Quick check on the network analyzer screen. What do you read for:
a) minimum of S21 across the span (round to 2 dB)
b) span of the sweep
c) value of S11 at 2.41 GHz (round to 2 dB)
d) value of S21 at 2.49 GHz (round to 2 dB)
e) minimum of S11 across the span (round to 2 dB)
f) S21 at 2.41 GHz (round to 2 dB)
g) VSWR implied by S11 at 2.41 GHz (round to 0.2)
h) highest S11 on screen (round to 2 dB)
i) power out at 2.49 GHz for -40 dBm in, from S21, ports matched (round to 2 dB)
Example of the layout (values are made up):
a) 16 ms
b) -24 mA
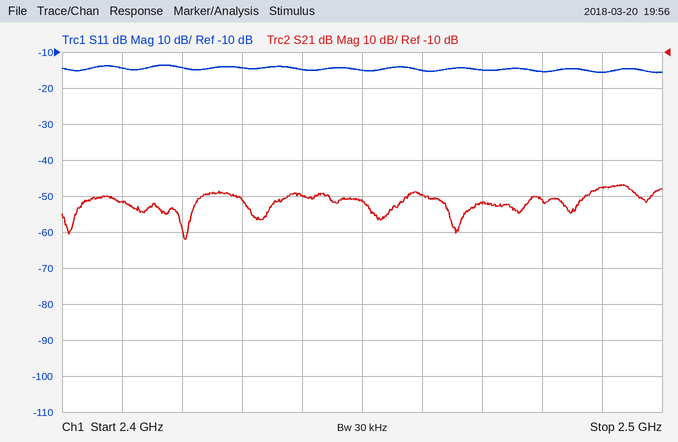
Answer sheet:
a) -62 dB
b) 100 MHz
c) -14 dB
d) -48 dB
e) -16 dB
f) -52 dB
g) 1.4
h) -14 dB
i) -88 dBm
